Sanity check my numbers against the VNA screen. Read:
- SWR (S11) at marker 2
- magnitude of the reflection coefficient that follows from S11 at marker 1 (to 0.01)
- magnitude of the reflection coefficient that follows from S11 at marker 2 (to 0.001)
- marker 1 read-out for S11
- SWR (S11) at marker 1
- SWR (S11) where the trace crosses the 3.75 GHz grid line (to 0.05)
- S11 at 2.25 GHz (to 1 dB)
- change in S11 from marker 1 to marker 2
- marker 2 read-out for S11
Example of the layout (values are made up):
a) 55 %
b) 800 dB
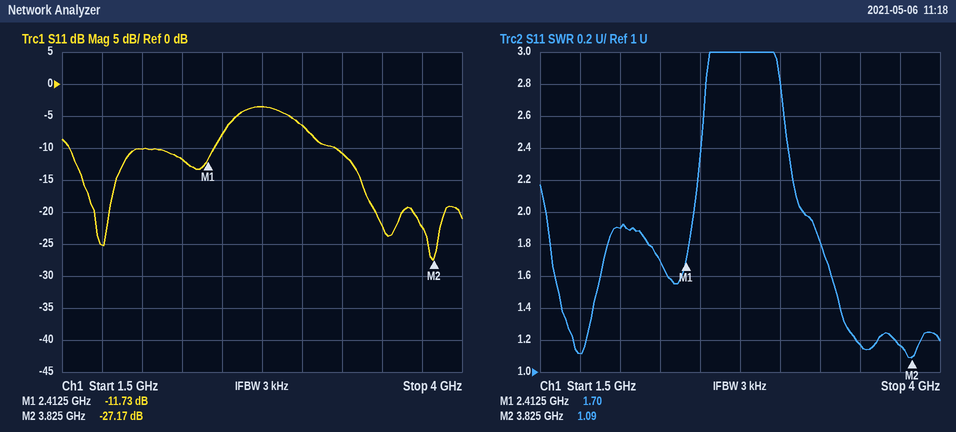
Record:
a) 1.09
b) 0.26
c) 0.044
d) -11.73 dB
e) 1.70
f) 1.15
g) -12 dB
h) -15.44 dB
i) -27.17 dB
